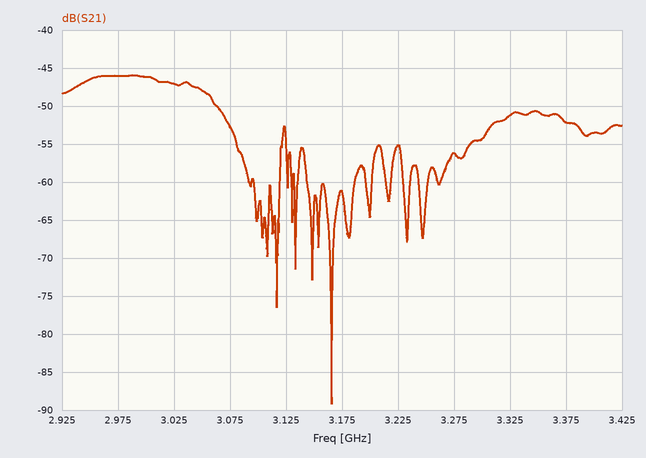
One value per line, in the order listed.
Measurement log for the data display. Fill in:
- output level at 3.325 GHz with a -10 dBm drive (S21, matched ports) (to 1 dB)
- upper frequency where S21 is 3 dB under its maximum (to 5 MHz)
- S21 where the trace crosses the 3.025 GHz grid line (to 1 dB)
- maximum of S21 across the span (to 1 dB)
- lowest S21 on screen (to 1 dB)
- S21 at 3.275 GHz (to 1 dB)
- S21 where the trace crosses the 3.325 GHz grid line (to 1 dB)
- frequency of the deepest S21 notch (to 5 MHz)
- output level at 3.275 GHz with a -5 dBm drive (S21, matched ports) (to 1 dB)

-61 dBm
3.060 GHz
-47 dB
-46 dB
-89 dB
-56 dB
-51 dB
3.165 GHz
-61 dBm
